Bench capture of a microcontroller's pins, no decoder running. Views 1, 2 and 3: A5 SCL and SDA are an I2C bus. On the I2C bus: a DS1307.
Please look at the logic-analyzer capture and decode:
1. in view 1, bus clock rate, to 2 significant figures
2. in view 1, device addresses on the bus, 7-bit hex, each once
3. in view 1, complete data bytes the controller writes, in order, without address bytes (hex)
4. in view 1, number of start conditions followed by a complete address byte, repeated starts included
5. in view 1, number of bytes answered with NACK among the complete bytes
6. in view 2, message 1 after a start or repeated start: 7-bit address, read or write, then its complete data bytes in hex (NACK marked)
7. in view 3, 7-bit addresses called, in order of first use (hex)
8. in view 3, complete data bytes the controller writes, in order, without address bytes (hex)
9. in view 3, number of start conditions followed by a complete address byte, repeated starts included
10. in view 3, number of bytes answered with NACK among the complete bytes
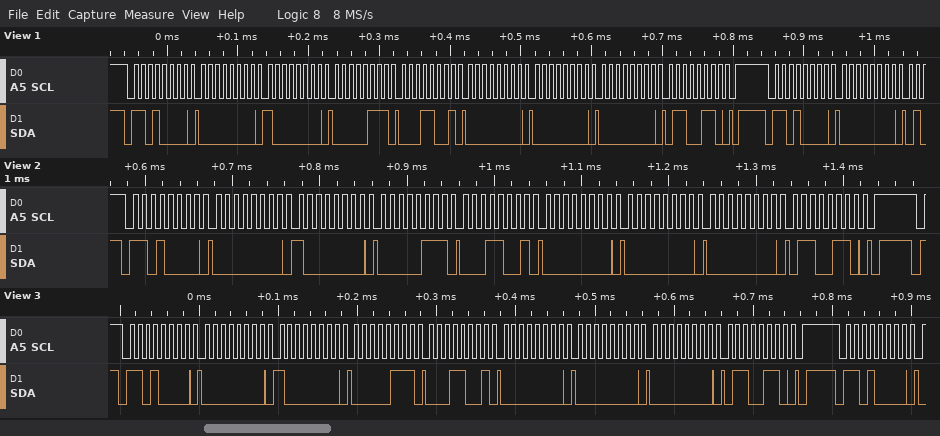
100 kHz
0x68
00 80 07 19 00 00 00 66 00
2
0
0x68 write: 00 80 07 19 00 00 00 66
0x68
00 80 07 19 00 00 00 66
2
0
